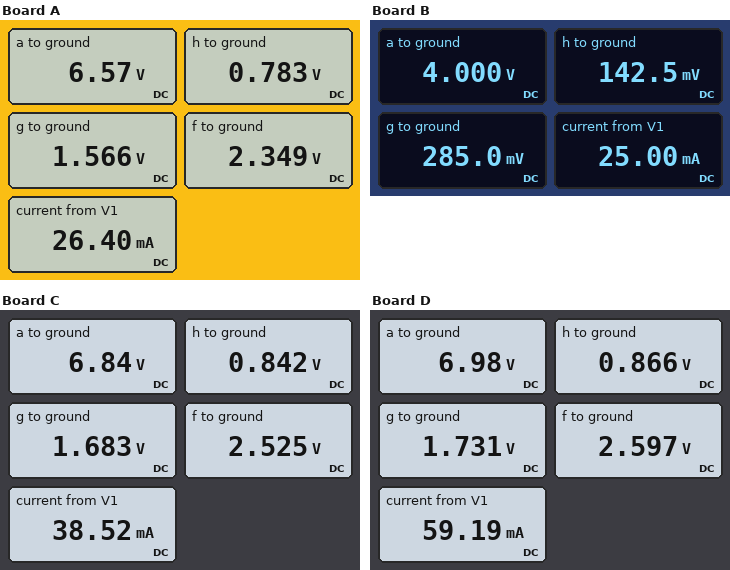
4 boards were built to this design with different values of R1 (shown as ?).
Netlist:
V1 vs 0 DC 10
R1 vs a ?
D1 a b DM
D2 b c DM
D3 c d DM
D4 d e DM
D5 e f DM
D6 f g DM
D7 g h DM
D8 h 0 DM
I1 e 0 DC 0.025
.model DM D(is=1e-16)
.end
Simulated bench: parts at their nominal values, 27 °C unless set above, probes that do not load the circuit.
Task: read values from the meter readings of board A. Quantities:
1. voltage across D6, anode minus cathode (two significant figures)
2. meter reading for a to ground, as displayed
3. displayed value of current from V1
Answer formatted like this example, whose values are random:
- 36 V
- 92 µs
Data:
- 780 mV
- 6.57 V
- 26.40 mA
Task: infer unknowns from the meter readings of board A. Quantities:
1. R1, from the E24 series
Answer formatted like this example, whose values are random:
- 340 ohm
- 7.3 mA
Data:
- 130 Ω
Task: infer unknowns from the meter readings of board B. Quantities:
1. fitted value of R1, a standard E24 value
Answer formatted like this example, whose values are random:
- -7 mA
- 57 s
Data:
- 240 Ω
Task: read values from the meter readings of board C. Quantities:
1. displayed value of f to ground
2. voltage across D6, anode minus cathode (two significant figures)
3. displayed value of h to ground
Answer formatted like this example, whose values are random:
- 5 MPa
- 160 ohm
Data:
- 2.525 V
- 840 mV
- 0.842 V
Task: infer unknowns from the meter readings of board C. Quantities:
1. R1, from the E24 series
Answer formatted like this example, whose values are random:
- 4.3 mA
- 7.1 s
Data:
- 82 Ω
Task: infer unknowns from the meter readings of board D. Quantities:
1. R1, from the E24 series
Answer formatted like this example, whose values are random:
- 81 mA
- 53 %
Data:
- 51 Ω
